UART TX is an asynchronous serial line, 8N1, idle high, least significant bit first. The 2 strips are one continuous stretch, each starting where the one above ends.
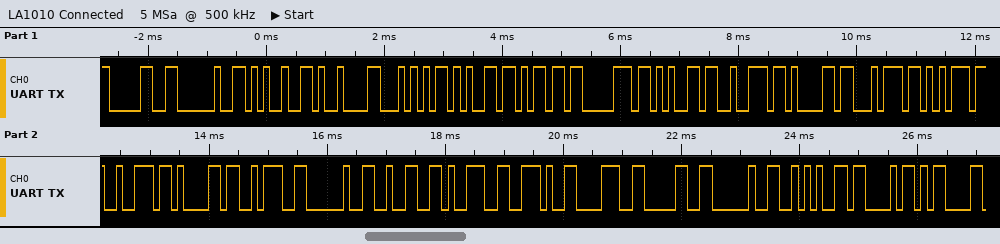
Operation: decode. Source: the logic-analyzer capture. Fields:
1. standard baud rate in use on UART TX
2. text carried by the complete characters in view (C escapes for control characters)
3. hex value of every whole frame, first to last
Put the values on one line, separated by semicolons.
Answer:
9600 baud; "0 %\tTemperatura: 29.80 *C\r"; 30 20 25 09 54 65 6D 70 65 72 61 74 75 72 61 3A 20 32 39 2E 38 30 20 2A 43 0D
